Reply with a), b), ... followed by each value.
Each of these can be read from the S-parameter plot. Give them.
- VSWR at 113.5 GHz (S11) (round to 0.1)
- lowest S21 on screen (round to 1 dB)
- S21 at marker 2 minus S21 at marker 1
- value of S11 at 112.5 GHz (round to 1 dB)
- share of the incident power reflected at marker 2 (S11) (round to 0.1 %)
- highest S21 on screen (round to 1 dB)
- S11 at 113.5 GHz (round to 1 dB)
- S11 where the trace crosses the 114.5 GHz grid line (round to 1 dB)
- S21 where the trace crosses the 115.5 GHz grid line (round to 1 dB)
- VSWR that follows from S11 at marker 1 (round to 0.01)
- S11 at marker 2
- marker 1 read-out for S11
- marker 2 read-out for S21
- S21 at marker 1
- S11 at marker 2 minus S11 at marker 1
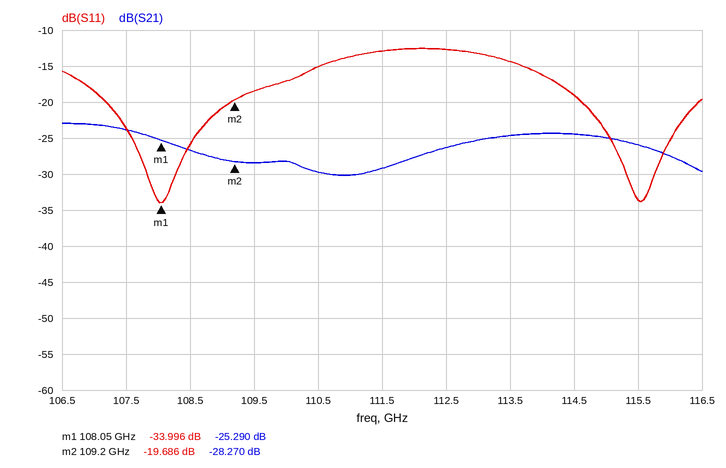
a) 1.5
b) -30 dB
c) -2.980 dB
d) -13 dB
e) 1.1 %
f) -23 dB
g) -14 dB
h) -19 dB
i) -26 dB
j) 1.04
k) -19.686 dB
l) -33.996 dB
m) -28.270 dB
n) -25.290 dB
o) 14.310 dB
